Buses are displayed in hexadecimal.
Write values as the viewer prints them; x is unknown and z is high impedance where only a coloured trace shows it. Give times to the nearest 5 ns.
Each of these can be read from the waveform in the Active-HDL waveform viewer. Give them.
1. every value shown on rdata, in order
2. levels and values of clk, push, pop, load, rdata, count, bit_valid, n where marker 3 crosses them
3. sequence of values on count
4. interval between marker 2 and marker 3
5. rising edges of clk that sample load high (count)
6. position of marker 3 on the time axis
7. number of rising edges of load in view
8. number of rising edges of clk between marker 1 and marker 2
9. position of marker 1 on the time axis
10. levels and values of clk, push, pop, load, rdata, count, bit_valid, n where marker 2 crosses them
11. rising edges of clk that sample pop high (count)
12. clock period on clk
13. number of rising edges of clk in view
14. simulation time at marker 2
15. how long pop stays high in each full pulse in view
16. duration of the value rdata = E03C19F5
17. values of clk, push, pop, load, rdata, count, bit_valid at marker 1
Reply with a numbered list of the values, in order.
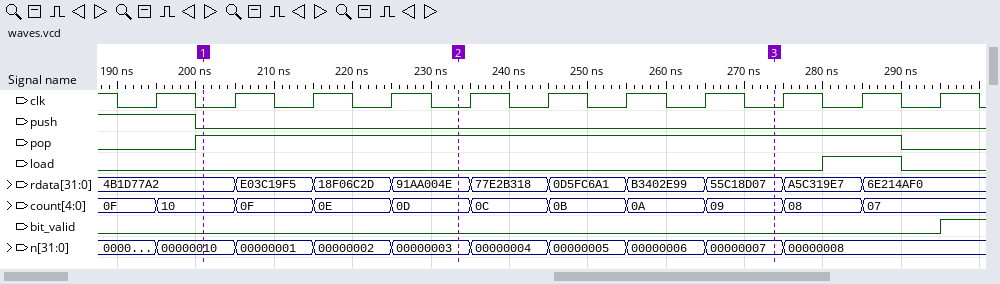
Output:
1. 4B1D77A2, E03C19F5, 18F06C2D, 91AA004E, 77E2B318, 0D5FC6A1, B3402E99, 55C18D07, A5C319E7, 6E214AF0
2. clk=0, push=0, pop=1, load=0, rdata=55C18D07, count=09, bit_valid=0, n=00000007
3. 0F, 10, 0F, 0E, 0D, 0C, 0B, 0A, 09, 08, 07
4. 40 ns
5. 1
6. 275 ns
7. 1
8. 3
9. 200 ns
10. clk=0, push=0, pop=1, load=0, rdata=91AA004E, count=0D, bit_valid=0, n=00000003
11. 9
12. 10 ns
13. 11
14. 235 ns
15. 90 ns
16. 10 ns
17. clk=0, push=0, pop=1, load=0, rdata=4B1D77A2, count=10, bit_valid=0
